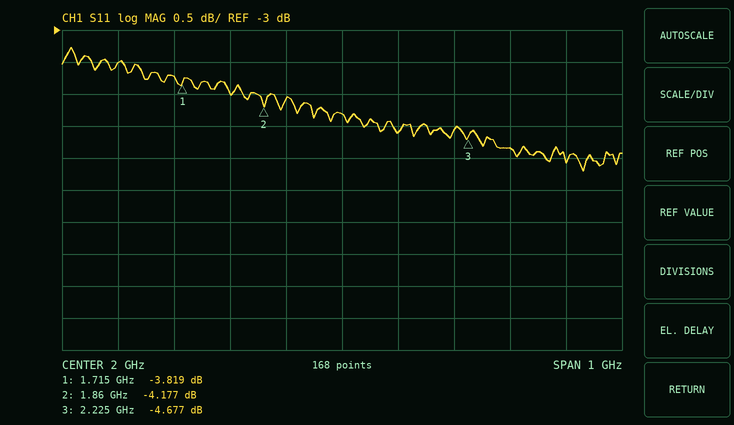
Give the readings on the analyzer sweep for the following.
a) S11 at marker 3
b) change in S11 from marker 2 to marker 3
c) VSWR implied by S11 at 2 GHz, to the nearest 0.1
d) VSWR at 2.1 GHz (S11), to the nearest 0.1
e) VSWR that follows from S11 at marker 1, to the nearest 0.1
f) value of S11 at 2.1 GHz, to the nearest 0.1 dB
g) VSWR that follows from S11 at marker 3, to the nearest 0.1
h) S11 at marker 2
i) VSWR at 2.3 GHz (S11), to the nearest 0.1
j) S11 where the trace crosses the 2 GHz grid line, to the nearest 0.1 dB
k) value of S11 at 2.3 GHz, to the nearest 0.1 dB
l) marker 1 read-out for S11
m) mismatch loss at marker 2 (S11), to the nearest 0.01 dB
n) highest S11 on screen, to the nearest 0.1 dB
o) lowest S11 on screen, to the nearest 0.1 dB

-4.677 dB
-0.500 dB
4.1
3.9
4.6
-4.6 dB
3.8
-4.177 dB
3.7
-4.3 dB
-4.8 dB
-3.819 dB
2.09 dB
-3.3 dB
-5.2 dB
